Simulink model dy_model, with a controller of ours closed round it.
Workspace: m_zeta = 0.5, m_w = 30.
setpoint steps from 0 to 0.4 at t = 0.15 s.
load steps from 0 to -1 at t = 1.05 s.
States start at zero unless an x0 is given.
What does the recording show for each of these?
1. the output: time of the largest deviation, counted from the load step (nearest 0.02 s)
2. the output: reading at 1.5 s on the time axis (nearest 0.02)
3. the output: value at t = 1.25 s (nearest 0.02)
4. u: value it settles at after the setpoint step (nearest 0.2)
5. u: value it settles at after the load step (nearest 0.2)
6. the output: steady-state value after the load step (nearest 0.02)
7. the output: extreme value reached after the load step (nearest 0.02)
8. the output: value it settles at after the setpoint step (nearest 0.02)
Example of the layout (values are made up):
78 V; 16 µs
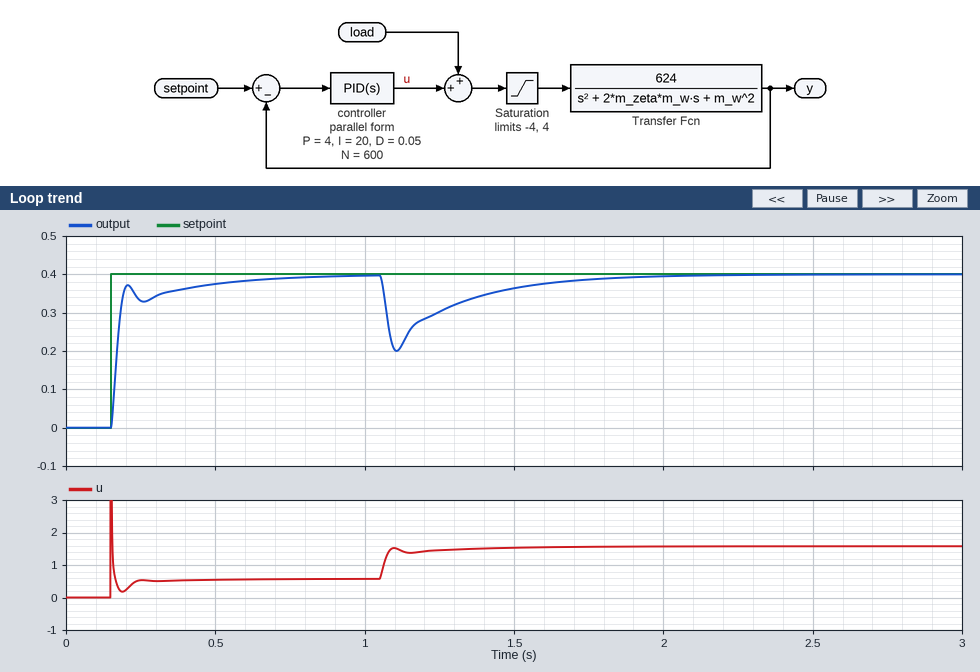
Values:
0.06 s; 0.36; 0.30; 0.6; 1.6; 0.40; 0.20; 0.40
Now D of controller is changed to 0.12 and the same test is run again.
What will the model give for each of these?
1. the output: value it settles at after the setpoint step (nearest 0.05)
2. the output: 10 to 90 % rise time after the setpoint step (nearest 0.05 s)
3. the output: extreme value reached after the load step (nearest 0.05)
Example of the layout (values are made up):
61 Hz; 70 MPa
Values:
0.40; 0.20 s; 0.25
